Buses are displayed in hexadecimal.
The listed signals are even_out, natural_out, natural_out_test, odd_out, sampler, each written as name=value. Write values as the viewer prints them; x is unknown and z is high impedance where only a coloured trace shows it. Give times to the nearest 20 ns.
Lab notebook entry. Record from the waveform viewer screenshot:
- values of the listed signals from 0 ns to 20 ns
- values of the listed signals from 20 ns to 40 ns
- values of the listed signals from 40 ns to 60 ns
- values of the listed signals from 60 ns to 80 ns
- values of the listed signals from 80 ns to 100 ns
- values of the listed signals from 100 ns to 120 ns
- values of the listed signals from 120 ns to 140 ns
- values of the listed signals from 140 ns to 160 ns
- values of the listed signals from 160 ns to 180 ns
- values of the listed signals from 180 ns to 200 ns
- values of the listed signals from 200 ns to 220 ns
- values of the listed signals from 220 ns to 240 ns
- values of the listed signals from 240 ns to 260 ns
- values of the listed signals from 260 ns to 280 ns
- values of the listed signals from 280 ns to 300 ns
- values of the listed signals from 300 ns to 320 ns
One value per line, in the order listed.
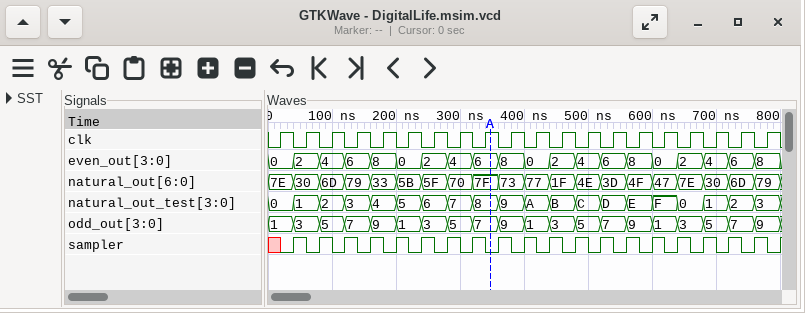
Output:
even_out=0, natural_out=7E, natural_out_test=0, odd_out=1, sampler=x
even_out=0, natural_out=7E, natural_out_test=0, odd_out=1, sampler=0
even_out=2, natural_out=30, natural_out_test=1, odd_out=3, sampler=1
even_out=2, natural_out=30, natural_out_test=1, odd_out=3, sampler=0
even_out=4, natural_out=6D, natural_out_test=2, odd_out=5, sampler=1
even_out=4, natural_out=6D, natural_out_test=2, odd_out=5, sampler=0
even_out=6, natural_out=79, natural_out_test=3, odd_out=7, sampler=1
even_out=6, natural_out=79, natural_out_test=3, odd_out=7, sampler=0
even_out=8, natural_out=33, natural_out_test=4, odd_out=9, sampler=1
even_out=8, natural_out=33, natural_out_test=4, odd_out=9, sampler=0
even_out=0, natural_out=5B, natural_out_test=5, odd_out=1, sampler=1
even_out=0, natural_out=5B, natural_out_test=5, odd_out=1, sampler=0
even_out=2, natural_out=5F, natural_out_test=6, odd_out=3, sampler=1
even_out=2, natural_out=5F, natural_out_test=6, odd_out=3, sampler=0
even_out=4, natural_out=70, natural_out_test=7, odd_out=5, sampler=1
even_out=4, natural_out=70, natural_out_test=7, odd_out=5, sampler=0
